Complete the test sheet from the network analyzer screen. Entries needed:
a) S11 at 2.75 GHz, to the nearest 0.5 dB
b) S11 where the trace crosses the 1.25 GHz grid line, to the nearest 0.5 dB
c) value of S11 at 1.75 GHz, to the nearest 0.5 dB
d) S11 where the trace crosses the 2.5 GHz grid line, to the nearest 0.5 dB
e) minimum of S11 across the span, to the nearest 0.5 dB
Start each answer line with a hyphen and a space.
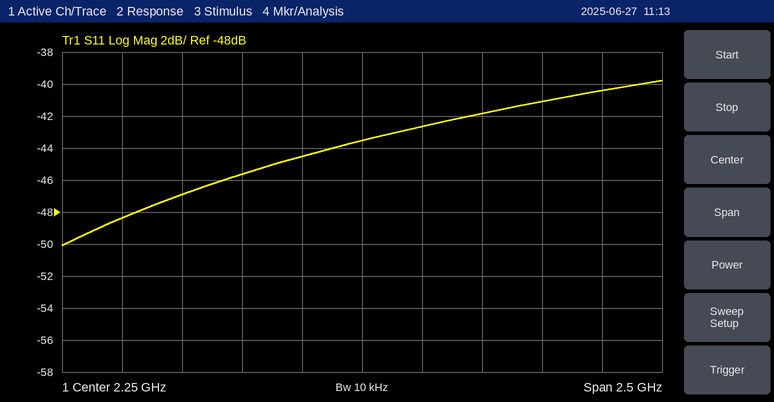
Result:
- -42.0 dB
- -48.5 dB
- -45.5 dB
- -42.5 dB
- -50.0 dB
